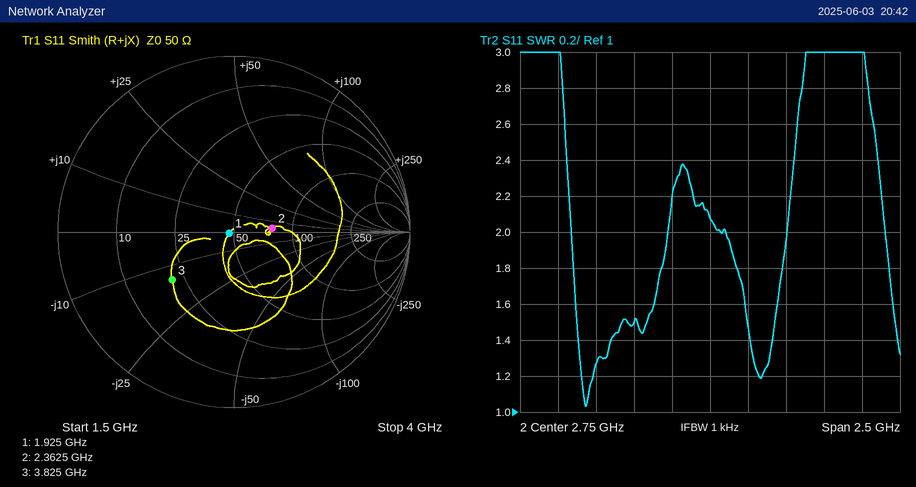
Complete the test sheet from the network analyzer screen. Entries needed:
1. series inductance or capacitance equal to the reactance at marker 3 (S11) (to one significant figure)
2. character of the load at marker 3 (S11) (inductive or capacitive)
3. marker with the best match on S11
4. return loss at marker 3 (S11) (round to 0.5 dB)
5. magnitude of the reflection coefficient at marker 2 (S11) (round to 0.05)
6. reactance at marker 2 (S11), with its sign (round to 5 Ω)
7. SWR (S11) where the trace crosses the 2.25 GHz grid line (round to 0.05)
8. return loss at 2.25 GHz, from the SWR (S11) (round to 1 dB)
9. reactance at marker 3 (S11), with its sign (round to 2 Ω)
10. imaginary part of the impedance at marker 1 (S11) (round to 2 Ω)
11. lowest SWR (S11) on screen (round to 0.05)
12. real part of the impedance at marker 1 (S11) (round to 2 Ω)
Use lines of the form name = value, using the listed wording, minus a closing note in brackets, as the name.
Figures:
series inductance or capacitance equal to the reactance at marker 3 (S11) = 3 pF
character of the load at marker 3 (S11) = capacitive
marker with the best match on S11 = marker 1
return loss at marker 3 (S11) = 7.0 dB
magnitude of the reflection coefficient at marker 2 (S11) = 0.20
reactance at marker 2 (S11), with its sign = +5 Ω
SWR (S11) where the trace crosses the 2.25 GHz grid line = 1.50
return loss at 2.25 GHz, from the SWR (S11) = 14 dB
reactance at marker 3 (S11), with its sign = -14 Ω
imaginary part of the impedance at marker 1 (S11) = 0 Ω
lowest SWR (S11) on screen = 1.05
real part of the impedance at marker 1 (S11) = 48 Ω
